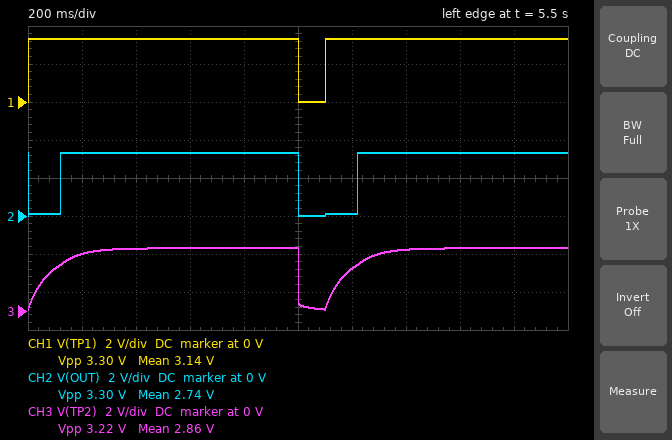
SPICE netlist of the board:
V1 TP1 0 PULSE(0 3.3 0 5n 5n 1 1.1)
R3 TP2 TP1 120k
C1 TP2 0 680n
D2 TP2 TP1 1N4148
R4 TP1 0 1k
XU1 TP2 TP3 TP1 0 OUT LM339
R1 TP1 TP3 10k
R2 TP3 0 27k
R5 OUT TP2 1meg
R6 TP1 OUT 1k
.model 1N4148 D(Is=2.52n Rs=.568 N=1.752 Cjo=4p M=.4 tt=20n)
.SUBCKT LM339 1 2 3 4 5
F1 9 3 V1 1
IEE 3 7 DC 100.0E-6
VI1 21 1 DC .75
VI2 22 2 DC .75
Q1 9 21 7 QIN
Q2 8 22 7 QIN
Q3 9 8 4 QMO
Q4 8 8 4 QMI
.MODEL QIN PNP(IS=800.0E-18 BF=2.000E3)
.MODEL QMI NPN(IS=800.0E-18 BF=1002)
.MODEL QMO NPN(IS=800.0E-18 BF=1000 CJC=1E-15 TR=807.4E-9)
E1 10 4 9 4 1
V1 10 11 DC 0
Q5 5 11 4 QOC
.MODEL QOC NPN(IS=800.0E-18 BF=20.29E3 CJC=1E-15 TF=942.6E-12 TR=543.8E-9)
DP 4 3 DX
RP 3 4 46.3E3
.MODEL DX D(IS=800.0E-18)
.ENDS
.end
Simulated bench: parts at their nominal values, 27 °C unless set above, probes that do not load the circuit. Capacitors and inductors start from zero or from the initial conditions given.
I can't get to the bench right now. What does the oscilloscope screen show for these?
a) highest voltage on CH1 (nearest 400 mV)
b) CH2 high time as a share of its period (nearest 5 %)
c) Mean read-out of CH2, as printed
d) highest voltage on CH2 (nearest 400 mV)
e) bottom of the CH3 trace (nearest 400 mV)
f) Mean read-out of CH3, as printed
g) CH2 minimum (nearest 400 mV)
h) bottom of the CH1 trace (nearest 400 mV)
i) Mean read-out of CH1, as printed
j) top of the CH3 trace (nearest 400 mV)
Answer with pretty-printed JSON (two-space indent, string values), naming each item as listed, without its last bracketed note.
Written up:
{
  "highest voltage on CH1": "3.2 V",
  "CH2 high time as a share of its period": "80 %",
  "Mean read-out of CH2, as printed": "2.74 V",
  "highest voltage on CH2": "3.2 V",
  "bottom of the CH3 trace": "0 V",
  "Mean read-out of CH3, as printed": "2.86 V",
  "CH2 minimum": "0 V",
  "bottom of the CH1 trace": "0 V",
  "Mean read-out of CH1, as printed": "3.14 V",
  "top of the CH3 trace": "3.2 V"
}
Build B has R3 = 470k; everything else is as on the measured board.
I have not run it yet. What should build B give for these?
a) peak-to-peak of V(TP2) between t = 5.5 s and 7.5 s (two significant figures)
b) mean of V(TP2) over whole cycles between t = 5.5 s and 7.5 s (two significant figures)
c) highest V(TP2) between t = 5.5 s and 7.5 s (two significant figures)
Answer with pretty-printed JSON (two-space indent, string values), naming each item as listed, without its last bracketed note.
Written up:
{
  "peak-to-peak of V(TP2) between t = 5.5 s and 7.5 s": "2.1 V",
  "mean of V(TP2) over whole cycles between t = 5.5 s and 7.5 s": "1.7 V",
  "highest V(TP2) between t = 5.5 s and 7.5 s": "2.3 V"
}
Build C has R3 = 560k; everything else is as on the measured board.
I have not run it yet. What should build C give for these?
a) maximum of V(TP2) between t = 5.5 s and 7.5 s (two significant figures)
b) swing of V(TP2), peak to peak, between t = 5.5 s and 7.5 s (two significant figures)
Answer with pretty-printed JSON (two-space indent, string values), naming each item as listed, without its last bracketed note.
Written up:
{
  "maximum of V(TP2) between t = 5.5 s and 7.5 s": "2.1 V",
  "swing of V(TP2), peak to peak, between t = 5.5 s and 7.5 s": "2.0 V"
}
